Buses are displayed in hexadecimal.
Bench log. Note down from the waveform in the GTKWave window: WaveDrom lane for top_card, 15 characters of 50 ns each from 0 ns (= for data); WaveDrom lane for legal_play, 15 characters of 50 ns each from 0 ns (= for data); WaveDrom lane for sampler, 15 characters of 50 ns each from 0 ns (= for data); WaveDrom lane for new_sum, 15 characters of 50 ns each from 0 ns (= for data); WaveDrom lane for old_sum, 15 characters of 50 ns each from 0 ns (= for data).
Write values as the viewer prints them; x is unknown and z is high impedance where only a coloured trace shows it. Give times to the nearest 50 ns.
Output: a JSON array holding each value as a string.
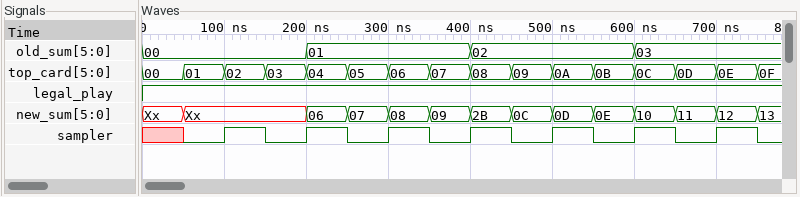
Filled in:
["{name: 'top_card', wave: '===============', data: '00 01 02 03 04 05 06 07 08 09 0A 0B 0C 0D 0E'}", "{name: 'legal_play', wave: '1..............'}", "{name: 'sampler', wave: 'x01010101010101'}", "{name: 'new_sum', wave: '==..===========', data: 'Xx Xx 06 07 08 09 2B 0C 0D 0E 10 11 12'}", "{name: 'old_sum', wave: '=...=...=...=..', data: '00 01 02 03'}"]
